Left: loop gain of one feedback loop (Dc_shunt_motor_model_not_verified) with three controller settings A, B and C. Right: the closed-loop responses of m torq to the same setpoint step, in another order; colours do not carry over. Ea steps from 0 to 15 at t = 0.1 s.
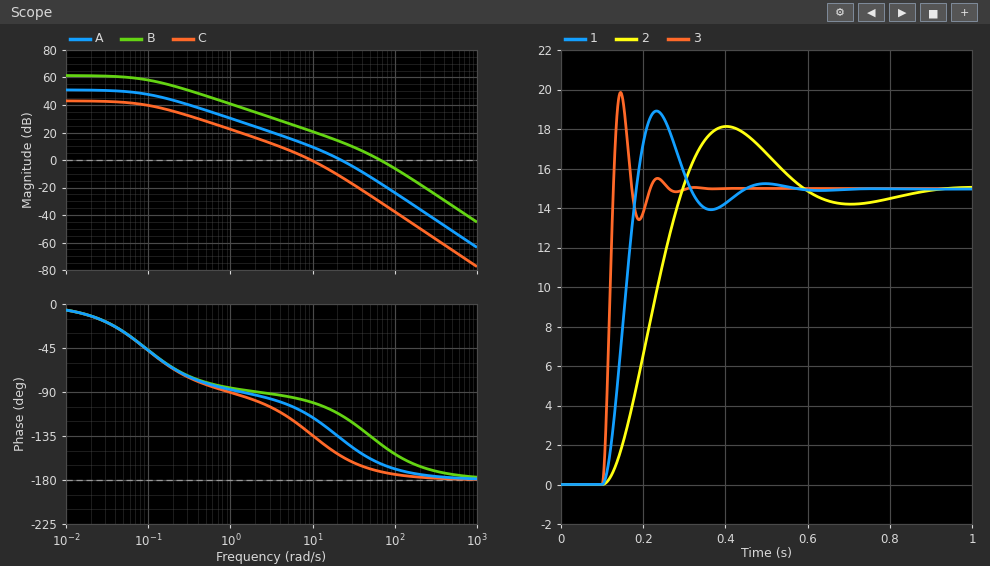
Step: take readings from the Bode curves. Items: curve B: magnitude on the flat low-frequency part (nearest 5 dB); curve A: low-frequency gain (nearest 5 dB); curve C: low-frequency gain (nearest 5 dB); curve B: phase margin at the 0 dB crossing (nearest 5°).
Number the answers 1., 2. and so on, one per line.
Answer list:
1. 60 dB
2. 50 dB
3. 45 dB
4. 35°
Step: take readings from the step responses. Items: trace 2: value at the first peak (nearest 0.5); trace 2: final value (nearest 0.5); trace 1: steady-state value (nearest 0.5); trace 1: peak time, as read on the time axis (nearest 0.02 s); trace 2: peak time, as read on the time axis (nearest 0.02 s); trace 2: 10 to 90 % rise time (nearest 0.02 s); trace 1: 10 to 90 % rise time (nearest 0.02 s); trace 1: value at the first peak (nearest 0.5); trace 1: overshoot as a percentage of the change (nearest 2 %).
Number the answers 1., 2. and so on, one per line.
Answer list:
1. 18.0
2. 15.0
3. 15.0
4. 0.24 s
5. 0.40 s
6. 0.14 s
7. 0.06 s
8. 19.0
9. 26 %
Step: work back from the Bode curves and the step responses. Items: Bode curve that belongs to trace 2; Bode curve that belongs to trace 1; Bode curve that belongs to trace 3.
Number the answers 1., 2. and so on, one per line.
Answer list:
1. C
2. A
3. B
